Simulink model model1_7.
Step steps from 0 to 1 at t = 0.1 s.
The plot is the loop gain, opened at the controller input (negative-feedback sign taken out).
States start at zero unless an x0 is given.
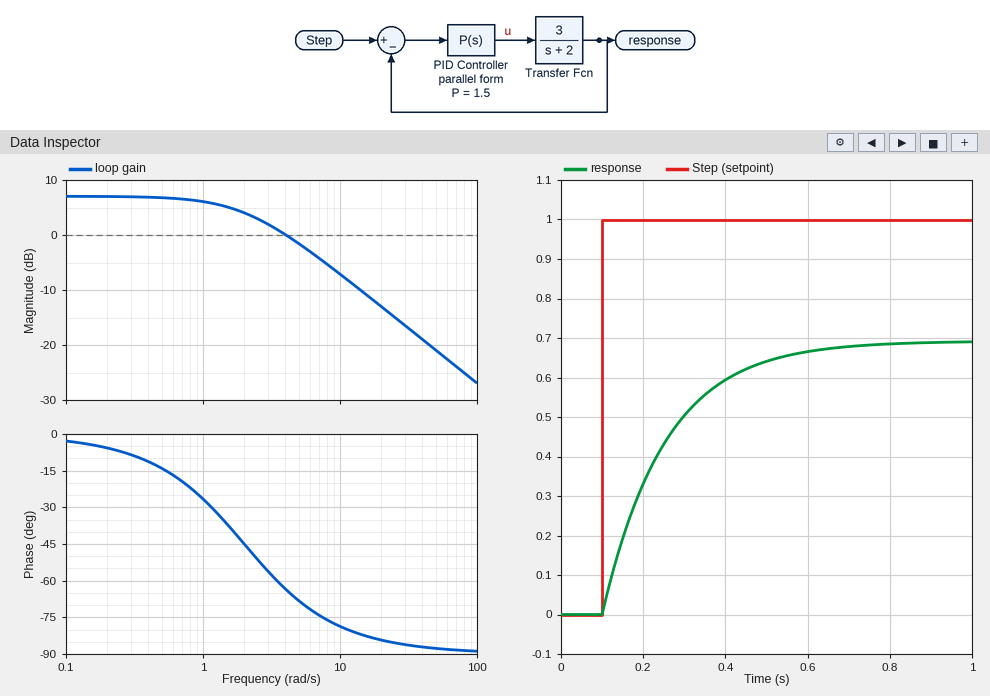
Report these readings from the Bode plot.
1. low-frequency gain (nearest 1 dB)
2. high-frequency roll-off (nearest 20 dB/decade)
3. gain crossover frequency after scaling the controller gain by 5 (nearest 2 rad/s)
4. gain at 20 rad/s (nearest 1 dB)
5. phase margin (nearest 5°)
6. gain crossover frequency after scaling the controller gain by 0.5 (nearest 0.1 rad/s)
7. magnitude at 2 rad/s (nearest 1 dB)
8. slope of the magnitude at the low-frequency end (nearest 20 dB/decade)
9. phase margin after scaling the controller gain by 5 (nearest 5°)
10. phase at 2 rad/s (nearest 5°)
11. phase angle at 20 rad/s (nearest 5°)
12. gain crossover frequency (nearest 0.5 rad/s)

7 dB
-20 dB/decade
22 rad/s
-13 dB
115°
1.0 rad/s
4 dB
0 dB/decade
95°
-45°
-85°
4.0 rad/s
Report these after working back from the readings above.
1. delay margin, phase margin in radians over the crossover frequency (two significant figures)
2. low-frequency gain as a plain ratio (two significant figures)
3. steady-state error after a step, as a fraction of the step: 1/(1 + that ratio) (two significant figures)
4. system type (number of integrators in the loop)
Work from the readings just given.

0.50 s
2.2
0.31
0
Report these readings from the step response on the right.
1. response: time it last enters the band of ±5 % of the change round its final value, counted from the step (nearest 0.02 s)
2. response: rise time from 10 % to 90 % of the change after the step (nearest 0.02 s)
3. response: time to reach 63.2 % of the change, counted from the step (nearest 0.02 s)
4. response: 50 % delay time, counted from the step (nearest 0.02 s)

0.46 s
0.34 s
0.16 s
0.10 s
